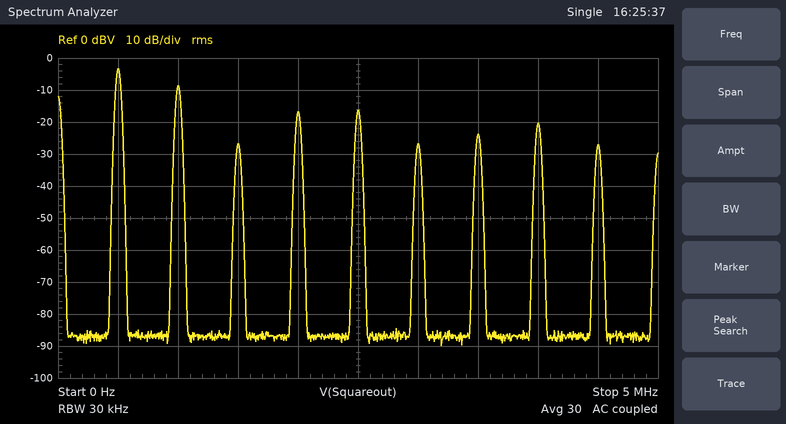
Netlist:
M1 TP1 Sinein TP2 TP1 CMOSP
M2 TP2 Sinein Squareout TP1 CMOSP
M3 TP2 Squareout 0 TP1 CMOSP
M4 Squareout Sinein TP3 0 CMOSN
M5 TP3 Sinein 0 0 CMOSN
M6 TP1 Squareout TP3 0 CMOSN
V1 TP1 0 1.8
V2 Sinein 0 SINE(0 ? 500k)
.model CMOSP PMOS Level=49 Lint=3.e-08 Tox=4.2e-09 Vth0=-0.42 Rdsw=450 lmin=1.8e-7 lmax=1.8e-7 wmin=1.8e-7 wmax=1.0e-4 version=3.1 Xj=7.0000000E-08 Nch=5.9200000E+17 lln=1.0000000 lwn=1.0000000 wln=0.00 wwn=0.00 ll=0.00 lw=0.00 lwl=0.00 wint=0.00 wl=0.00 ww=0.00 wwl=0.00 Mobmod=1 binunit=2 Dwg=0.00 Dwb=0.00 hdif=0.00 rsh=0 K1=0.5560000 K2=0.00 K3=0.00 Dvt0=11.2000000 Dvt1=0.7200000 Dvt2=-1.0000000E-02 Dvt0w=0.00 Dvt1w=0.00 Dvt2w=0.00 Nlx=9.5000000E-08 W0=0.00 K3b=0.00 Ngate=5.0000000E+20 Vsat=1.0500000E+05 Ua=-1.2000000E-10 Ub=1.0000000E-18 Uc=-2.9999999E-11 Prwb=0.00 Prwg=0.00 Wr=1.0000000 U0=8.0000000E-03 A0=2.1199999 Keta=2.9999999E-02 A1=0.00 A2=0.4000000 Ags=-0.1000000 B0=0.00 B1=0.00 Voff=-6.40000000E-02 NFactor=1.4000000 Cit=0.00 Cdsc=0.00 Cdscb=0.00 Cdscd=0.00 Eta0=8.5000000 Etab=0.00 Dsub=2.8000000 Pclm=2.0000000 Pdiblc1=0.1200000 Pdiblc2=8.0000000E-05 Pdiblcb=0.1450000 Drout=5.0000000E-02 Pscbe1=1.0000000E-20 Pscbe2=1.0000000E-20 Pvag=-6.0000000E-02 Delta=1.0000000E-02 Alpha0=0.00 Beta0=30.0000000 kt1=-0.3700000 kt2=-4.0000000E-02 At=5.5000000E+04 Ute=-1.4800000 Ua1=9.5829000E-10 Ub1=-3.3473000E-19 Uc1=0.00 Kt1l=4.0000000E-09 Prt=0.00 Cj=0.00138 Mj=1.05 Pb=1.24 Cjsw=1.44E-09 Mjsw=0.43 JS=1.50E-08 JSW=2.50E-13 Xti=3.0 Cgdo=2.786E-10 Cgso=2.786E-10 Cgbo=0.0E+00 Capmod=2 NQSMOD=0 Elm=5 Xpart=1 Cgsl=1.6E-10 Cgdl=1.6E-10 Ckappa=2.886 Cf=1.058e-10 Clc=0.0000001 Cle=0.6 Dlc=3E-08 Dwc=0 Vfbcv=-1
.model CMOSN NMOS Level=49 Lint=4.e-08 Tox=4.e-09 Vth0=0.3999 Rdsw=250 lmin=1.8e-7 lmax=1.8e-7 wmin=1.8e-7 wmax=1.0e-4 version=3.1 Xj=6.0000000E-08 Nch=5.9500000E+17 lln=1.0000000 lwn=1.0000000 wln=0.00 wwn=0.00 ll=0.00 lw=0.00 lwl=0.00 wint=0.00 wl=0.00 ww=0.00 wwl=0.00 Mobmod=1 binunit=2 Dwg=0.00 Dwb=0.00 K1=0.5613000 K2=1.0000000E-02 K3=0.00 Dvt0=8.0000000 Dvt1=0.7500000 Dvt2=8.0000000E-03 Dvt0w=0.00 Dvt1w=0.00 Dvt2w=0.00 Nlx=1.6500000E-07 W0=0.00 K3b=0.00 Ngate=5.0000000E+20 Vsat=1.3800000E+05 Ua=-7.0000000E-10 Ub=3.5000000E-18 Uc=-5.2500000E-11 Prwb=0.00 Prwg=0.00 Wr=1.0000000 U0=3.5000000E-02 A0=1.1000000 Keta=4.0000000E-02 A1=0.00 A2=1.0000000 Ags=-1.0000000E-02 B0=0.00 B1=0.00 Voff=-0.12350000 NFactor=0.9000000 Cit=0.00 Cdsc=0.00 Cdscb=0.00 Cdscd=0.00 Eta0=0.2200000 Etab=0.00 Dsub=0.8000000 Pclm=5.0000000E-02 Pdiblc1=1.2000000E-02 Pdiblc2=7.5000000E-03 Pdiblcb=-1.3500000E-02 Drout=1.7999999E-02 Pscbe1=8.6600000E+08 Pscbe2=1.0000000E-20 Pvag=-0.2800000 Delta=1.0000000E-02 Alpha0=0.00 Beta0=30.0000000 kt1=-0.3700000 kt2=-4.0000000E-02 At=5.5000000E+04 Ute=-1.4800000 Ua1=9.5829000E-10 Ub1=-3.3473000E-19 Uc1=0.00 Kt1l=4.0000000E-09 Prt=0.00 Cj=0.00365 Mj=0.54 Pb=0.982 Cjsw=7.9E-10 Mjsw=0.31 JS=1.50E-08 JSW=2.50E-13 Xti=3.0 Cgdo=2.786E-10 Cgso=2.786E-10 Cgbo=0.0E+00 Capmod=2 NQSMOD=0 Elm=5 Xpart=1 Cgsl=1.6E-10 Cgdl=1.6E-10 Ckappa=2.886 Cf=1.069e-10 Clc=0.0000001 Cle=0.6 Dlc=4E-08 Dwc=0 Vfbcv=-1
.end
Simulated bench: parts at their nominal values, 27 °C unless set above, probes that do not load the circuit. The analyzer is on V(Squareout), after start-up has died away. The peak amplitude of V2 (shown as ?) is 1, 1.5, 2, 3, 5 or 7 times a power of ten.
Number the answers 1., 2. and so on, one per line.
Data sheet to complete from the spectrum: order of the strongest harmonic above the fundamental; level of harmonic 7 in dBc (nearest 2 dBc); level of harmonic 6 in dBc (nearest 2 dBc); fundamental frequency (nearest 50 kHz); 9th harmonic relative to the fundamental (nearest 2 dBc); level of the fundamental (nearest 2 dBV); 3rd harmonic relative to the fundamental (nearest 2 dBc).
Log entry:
1. 2
2. -20 dBc
3. -24 dBc
4. 500 kHz
5. -24 dBc
6. -4 dBV
7. -24 dBc
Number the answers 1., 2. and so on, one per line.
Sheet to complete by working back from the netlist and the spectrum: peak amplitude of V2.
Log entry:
1. 1.5 V
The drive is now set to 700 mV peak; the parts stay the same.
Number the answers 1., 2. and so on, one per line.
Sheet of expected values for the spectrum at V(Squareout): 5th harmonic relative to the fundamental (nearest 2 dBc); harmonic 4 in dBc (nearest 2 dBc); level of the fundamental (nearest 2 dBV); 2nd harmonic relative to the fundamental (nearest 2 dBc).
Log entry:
1. -36 dBc
2. -22 dBc
3. -42 dBV
4. -50 dBc
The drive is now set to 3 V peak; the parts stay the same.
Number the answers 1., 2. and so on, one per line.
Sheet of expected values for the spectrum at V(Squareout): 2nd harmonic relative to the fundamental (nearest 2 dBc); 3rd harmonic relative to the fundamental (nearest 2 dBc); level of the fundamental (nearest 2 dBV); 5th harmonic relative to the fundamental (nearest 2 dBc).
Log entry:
1. -12 dBc
2. -12 dBc
3. -2 dBV
4. -24 dBc
